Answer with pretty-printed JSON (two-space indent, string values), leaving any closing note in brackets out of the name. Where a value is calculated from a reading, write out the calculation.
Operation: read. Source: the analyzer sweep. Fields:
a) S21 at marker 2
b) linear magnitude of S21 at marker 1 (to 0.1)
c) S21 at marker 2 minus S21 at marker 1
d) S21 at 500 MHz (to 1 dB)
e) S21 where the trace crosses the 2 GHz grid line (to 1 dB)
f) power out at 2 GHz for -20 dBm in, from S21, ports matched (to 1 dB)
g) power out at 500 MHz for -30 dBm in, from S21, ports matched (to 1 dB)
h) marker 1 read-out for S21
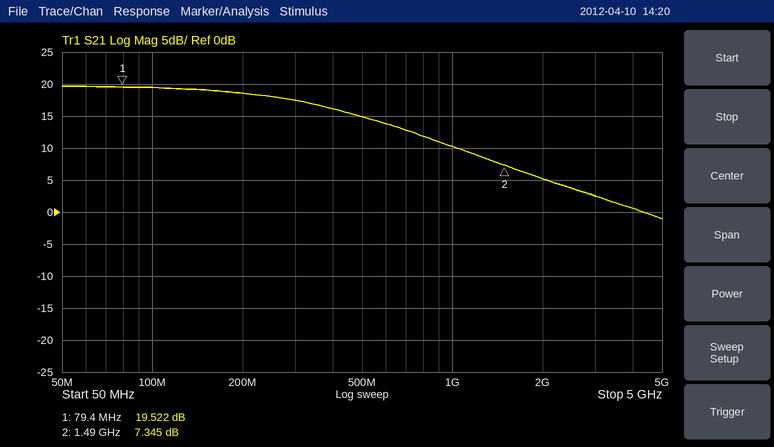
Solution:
{
  "S21 at marker 2": "7.345 dB",
  "linear magnitude of S21 at marker 1": "10^(19.522/20) ≈ 9.5",
  "S21 at marker 2 minus S21 at marker 1": "7.345 − (19.522) = -12.177 dB",
  "S21 at 500 MHz": "15 dB",
  "S21 where the trace crosses the 2 GHz grid line": "5 dB",
  "power out at 2 GHz for -20 dBm in, from S21, ports matched": "-20 dBm + (5 dB) = -15 dBm",
  "power out at 500 MHz for -30 dBm in, from S21, ports matched": "-30 dBm + (15 dB) = -15 dBm",
  "marker 1 read-out for S21": "19.522 dB"
}
